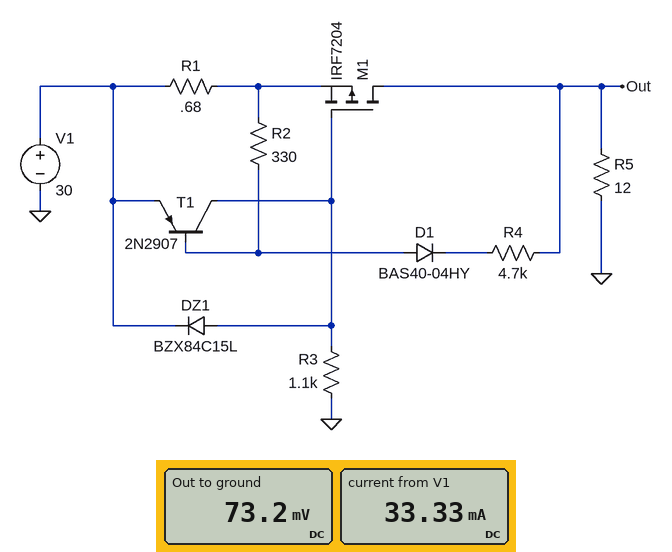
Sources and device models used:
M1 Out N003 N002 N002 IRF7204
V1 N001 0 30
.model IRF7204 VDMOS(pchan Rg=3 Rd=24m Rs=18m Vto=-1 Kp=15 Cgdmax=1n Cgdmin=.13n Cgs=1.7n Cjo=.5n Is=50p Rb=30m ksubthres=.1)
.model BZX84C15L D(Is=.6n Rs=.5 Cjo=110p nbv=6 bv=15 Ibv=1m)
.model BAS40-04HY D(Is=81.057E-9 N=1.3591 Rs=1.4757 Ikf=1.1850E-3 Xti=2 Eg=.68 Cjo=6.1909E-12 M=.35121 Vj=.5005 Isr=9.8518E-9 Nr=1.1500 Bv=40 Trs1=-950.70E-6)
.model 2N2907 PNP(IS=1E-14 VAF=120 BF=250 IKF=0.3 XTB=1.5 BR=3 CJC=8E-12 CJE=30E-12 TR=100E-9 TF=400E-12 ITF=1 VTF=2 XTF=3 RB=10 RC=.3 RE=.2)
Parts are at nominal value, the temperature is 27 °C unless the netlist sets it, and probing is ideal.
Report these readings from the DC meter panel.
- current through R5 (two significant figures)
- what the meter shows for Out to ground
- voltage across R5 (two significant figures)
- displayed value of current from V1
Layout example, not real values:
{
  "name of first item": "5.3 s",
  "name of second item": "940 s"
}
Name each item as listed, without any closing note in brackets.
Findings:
{
  "current through R5": "6.1 mA",
  "what the meter shows for Out to ground": "73.2 mV",
  "voltage across R5": "73 mV",
  "displayed value of current from V1": "33.33 mA"
}
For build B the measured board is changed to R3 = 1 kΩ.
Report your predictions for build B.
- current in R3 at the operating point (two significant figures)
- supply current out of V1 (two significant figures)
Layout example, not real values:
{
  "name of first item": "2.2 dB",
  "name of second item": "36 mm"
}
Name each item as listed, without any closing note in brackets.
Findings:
{
  "current in R3 at the operating point": "30 mA",
  "supply current out of V1": "36 mA"
}
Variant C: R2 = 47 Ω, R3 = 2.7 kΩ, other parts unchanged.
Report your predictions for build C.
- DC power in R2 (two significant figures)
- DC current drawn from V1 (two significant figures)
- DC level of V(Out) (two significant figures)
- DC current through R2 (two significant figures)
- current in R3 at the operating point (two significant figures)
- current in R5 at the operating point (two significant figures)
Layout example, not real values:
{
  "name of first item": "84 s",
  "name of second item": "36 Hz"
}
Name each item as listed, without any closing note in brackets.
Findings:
{
  "DC power in R2": "800 µW",
  "DC current drawn from V1": "780 mA",
  "DC level of V(Out)": "9.3 V",
  "DC current through R2": "4.1 mA",
  "current in R3 at the operating point": "10 mA",
  "current in R5 at the operating point": "770 mA"
}
